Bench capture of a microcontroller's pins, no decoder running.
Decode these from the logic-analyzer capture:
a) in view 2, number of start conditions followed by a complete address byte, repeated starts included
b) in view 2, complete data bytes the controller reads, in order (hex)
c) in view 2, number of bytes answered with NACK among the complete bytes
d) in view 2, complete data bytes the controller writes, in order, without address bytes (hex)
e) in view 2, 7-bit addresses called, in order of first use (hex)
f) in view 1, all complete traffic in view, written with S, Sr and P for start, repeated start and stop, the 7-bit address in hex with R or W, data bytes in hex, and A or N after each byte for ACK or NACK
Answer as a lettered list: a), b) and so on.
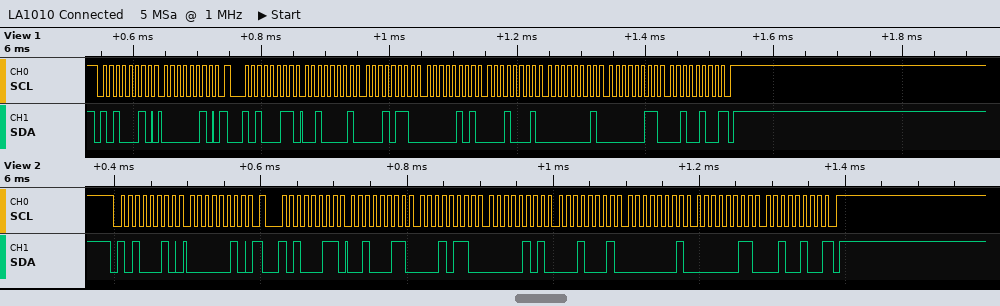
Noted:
a) 2
b) 23 16 05 11 01 03 24
c) 1
d) 02
e) 0x51
f) S 51W A 02 A Sr 51R A 21 A 16 A 05 A 11 A 01 A 03 A 24 N P
